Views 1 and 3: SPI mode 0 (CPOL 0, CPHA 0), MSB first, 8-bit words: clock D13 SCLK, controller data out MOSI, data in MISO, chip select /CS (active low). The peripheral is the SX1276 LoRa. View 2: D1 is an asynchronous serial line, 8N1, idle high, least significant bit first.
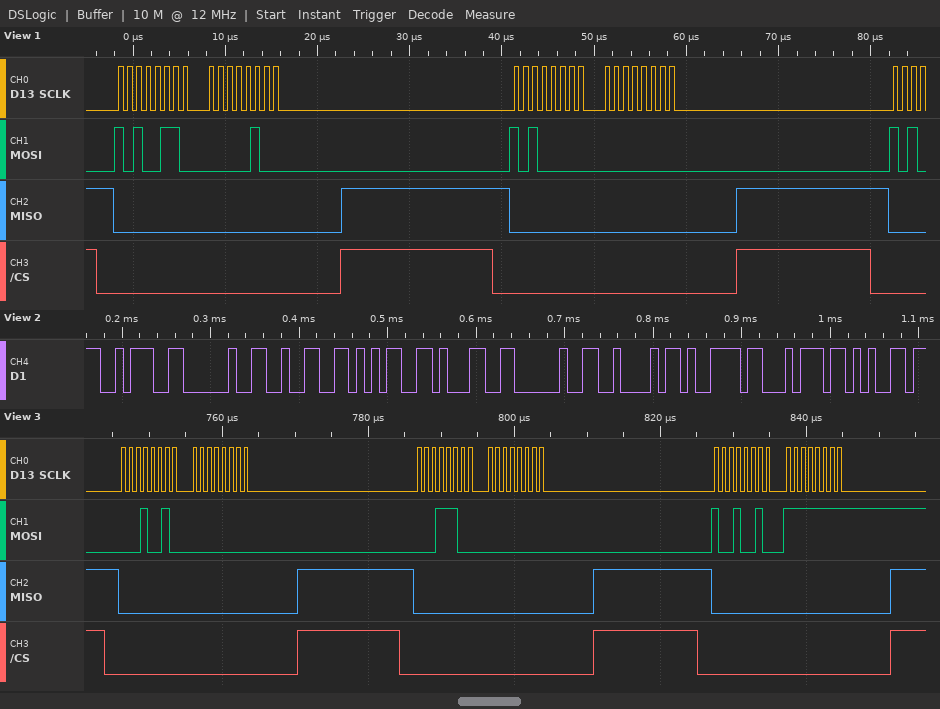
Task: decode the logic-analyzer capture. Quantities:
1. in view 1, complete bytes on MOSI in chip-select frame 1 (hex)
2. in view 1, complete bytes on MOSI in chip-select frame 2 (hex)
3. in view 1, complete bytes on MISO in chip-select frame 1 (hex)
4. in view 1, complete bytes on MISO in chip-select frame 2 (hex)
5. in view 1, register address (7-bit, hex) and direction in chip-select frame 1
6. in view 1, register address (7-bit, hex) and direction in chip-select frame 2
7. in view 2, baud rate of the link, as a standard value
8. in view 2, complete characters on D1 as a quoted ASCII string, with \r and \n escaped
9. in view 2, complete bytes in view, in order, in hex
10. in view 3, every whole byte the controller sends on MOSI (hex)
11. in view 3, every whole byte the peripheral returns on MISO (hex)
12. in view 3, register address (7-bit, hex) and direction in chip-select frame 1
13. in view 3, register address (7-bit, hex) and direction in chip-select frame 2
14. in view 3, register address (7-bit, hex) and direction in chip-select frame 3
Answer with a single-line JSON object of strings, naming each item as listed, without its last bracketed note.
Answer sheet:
{"in view 1, complete bytes on MOSI in chip-select frame 1": "A6 04", "in view 1, complete bytes on MOSI in chip-select frame 2": "A0 00", "in view 1, complete bytes on MISO in chip-select frame 1": "00 00", "in view 1, complete bytes on MISO in chip-select frame 2": "00 00", "in view 1, register address (7-bit, hex) and direction in chip-select frame 1": "0x26 write", "in view 1, register address (7-bit, hex) and direction in chip-select frame 2": "0x20 write", "in view 2, baud rate of the link, as a standard value": "115200 baud", "in view 2, complete characters on D1 as a quoted ASCII string, with \\r and \\n escaped": "\": 251 Byte\"", "in view 2, complete bytes in view, in order, in hex": "3A 20 32 35 31 20 42 79 74 65", "in view 3, every whole byte the controller sends on MOSI": "12 00 1C 00 92 FF", "in view 3, every whole byte the peripheral returns on MISO": "00 00 00 00 00 00", "in view 3, register address (7-bit, hex) and direction in chip-select frame 1": "0x12 read", "in view 3, register address (7-bit, hex) and direction in chip-select frame 2": "0x1C read", "in view 3, register address (7-bit, hex) and direction in chip-select frame 3": "0x12 write"}
